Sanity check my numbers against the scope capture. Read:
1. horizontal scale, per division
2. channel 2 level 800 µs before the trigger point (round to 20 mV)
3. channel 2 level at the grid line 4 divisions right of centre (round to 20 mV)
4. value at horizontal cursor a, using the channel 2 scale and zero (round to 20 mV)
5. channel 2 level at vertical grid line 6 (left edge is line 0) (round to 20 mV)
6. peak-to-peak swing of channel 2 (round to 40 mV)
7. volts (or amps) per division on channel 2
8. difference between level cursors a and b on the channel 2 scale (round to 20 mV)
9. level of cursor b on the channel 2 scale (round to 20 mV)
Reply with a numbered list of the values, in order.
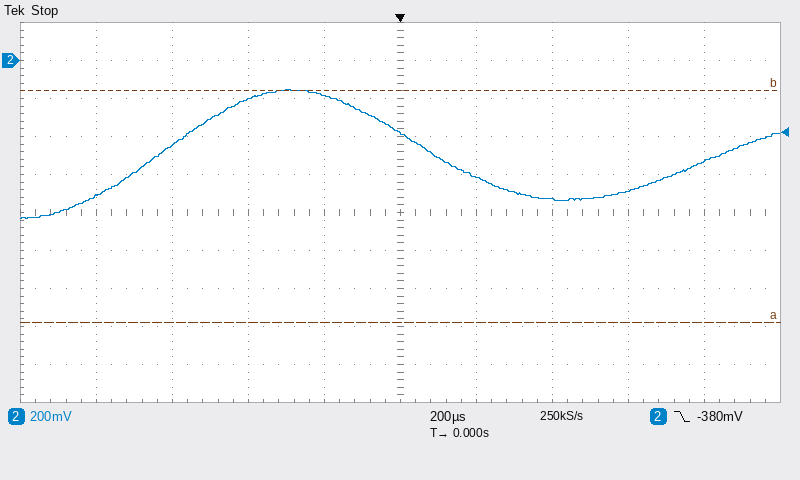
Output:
1. 200 µs
2. -720 mV
3. -540 mV
4. -1.38 V
5. -620 mV
6. 680 mV
7. 200 mV
8. 1.22 V
9. -160 mV
